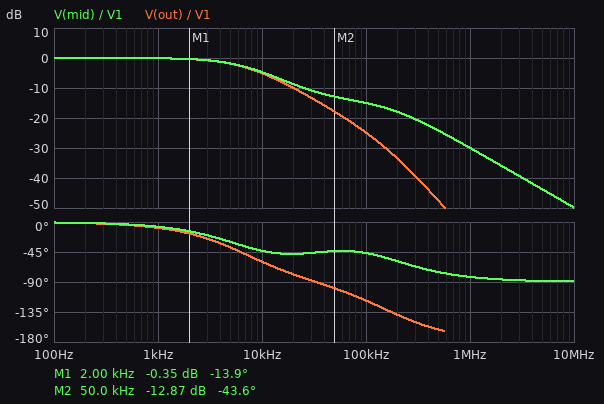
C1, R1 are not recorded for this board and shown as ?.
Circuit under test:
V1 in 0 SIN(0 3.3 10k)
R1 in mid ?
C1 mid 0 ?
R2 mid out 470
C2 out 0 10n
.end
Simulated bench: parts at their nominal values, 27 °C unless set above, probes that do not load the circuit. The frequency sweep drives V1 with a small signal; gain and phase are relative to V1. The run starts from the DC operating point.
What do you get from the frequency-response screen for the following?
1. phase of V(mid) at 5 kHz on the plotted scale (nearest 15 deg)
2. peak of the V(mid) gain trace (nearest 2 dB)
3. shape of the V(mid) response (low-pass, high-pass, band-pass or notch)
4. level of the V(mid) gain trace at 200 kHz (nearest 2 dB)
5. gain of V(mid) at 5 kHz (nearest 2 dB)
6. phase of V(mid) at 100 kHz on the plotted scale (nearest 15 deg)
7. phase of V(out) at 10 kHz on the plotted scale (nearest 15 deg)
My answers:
-30 deg
0 dB
low-pass
-18 dB
-2 dB
-45 deg
-60 deg
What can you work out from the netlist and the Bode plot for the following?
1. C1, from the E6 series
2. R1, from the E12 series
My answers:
3.3 nF
1.5 kΩ
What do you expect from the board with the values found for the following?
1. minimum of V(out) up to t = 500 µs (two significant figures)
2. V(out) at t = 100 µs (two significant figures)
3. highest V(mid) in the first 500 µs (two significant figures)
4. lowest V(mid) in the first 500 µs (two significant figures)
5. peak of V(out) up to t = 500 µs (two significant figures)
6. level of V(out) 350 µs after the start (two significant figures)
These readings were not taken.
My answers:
-1.8 V
-1.6 V
2.2 V
-1.9 V
2.1 V
1.6 V
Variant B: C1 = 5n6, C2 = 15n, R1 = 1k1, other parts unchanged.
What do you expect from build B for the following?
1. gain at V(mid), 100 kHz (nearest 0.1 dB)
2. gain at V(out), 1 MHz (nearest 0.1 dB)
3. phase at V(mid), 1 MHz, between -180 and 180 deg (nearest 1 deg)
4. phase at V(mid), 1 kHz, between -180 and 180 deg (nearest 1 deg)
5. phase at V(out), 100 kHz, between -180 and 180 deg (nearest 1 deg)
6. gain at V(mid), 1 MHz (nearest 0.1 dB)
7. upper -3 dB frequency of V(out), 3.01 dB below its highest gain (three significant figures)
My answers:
-14.7 dB
-64.7 dB
-85 deg
-8 deg
-131 deg
-31.8 dB
5.63 kHz
